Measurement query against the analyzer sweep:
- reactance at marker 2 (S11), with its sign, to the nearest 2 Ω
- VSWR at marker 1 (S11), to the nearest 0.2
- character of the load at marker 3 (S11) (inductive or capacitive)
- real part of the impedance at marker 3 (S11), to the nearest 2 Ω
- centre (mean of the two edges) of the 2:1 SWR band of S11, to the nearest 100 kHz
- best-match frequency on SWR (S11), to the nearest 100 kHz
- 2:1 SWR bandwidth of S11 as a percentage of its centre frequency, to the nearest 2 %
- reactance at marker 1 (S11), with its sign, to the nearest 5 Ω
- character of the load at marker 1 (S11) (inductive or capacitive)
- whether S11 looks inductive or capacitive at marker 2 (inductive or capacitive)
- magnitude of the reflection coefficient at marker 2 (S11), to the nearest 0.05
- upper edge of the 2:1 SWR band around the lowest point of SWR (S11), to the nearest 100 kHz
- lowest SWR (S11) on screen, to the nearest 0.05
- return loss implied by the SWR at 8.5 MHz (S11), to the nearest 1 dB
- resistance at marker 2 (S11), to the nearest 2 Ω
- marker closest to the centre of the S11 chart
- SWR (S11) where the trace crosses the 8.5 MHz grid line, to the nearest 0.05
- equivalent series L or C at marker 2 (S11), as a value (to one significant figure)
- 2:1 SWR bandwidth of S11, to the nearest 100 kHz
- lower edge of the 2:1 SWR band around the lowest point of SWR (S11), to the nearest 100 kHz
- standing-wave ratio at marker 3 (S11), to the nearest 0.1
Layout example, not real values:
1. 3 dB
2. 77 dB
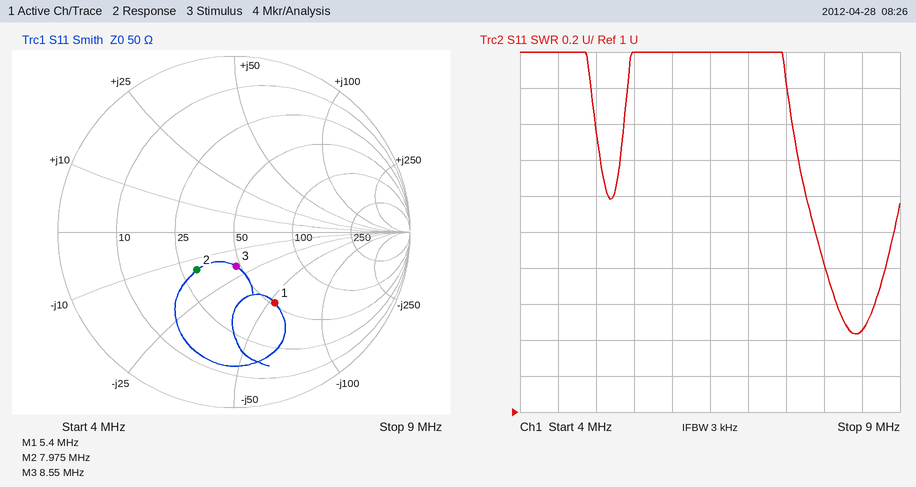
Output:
1. -14 Ω
2. 2.8
3. capacitive
4. 48 Ω
5. 8.4 MHz
6. 8.4 MHz
7. 12 %
8. -55 Ω
9. capacitive
10. capacitive
11. 0.30
12. 8.9 MHz
13. 1.45
14. 15 dB
15. 30 Ω
16. marker 3
17. 1.45
18. 1 nF
19. 1.0 MHz
20. 7.9 MHz
21. 1.5
